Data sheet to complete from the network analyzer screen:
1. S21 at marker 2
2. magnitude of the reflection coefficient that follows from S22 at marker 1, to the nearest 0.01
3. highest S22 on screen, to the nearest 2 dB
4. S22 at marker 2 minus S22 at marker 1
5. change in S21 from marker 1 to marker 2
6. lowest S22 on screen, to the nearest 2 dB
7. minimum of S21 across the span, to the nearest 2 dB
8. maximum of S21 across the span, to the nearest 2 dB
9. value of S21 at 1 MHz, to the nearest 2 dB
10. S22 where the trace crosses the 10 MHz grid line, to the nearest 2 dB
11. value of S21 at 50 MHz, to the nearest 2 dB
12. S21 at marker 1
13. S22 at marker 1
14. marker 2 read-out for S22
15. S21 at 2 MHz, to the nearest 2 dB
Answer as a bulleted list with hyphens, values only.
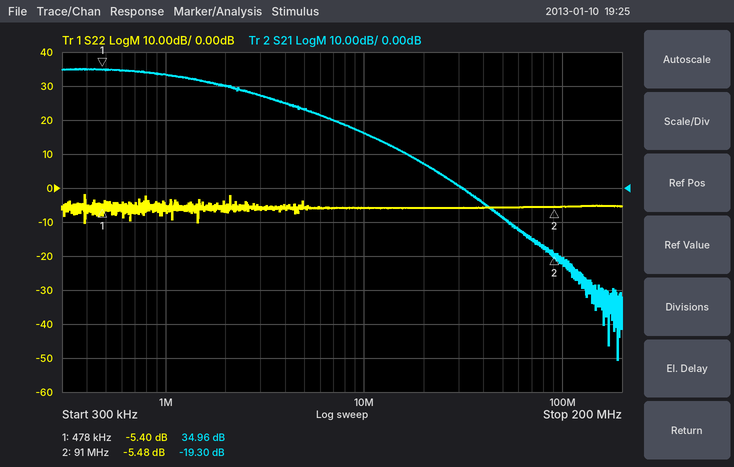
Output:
- -19.30 dB
- 0.54
- -2 dB
- -0.08 dB
- -54.26 dB
- -10 dB
- -50 dB
- 36 dB
- 34 dB
- -6 dB
- -8 dB
- 34.96 dB
- -5.40 dB
- -5.48 dB
- 30 dB
